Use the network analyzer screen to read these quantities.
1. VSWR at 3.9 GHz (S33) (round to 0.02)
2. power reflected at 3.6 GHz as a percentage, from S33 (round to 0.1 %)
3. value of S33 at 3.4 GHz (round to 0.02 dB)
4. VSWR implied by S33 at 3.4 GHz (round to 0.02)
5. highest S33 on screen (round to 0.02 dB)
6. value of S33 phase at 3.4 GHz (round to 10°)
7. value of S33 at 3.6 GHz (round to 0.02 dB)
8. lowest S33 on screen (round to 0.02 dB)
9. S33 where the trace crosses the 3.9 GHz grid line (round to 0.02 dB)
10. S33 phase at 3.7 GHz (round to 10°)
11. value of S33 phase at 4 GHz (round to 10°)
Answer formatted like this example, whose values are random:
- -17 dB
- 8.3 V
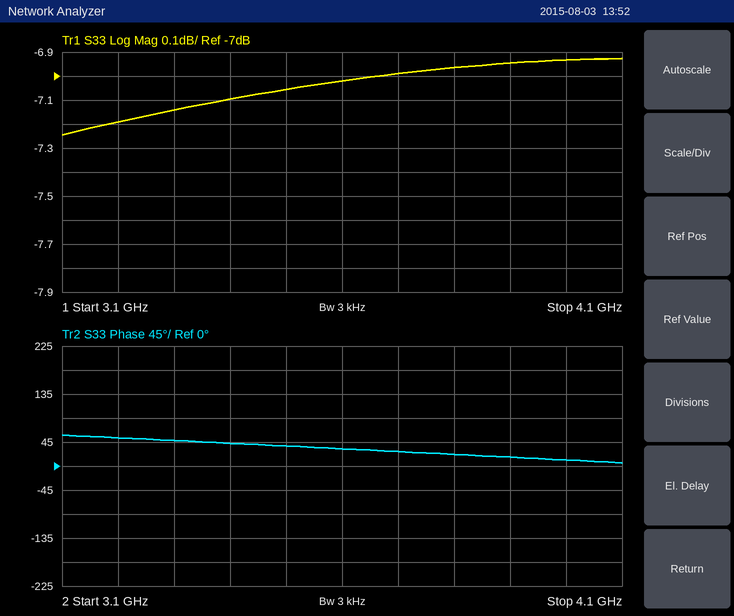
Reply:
- 2.64
- 19.9 %
- -7.10 dB
- 2.58
- -6.92 dB
- 40°
- -7.02 dB
- -7.24 dB
- -6.94 dB
- 30°
- 10°
